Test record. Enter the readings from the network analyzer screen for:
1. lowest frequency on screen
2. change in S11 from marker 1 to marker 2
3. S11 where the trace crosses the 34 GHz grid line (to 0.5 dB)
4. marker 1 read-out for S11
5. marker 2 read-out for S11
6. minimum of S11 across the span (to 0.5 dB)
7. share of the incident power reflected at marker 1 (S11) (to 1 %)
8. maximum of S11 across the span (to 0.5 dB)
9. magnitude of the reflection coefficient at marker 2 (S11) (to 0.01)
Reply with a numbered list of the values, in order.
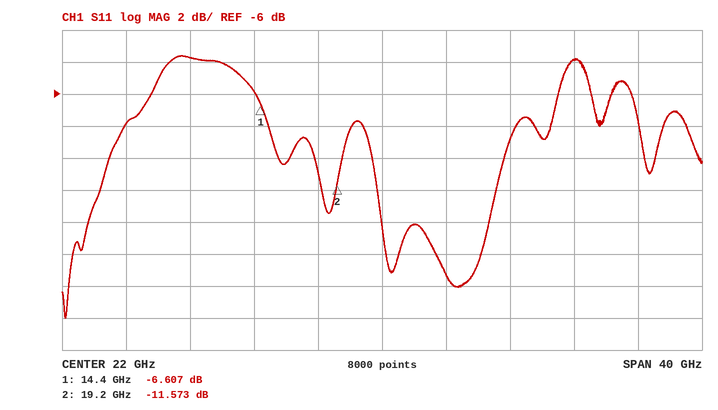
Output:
1. 2 GHz
2. -4.966 dB
3. -4.0 dB
4. -6.607 dB
5. -11.573 dB
6. -20.0 dB
7. 22 %
8. -3.5 dB
9. 0.26
